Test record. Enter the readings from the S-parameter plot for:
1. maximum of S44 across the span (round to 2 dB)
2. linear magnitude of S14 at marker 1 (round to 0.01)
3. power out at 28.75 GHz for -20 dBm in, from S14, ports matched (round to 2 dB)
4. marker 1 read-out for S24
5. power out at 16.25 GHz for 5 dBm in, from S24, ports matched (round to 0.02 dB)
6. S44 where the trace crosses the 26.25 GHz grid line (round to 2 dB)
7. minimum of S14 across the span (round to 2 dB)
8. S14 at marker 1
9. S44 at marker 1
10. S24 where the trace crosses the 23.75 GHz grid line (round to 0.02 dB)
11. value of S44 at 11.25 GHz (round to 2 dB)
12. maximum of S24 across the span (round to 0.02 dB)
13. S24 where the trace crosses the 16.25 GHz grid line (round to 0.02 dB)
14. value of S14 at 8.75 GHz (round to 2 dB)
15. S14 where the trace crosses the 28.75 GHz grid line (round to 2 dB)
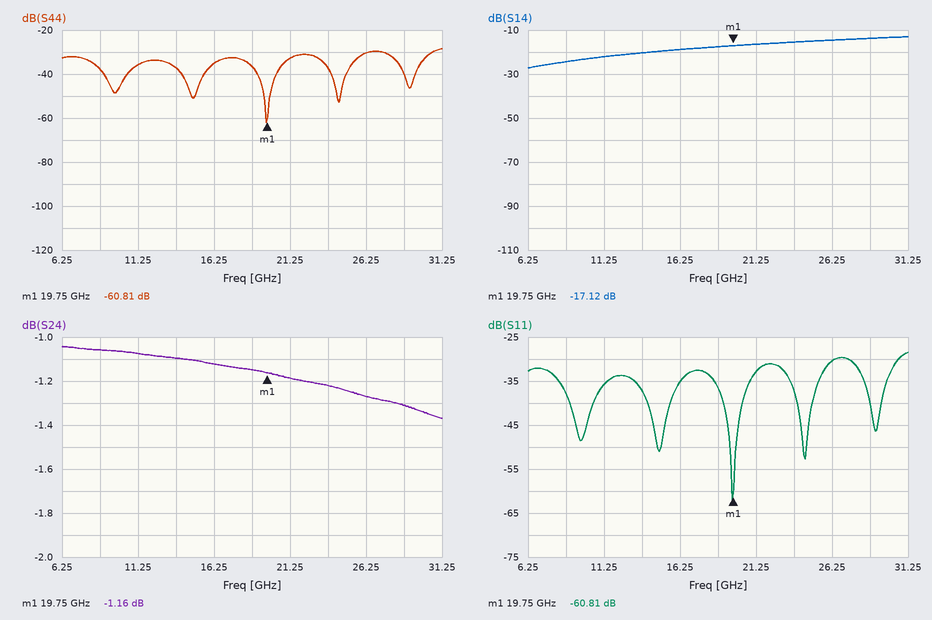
-28 dB
0.14
-34 dBm
-1.16 dB
3.88 dBm
-30 dB
-28 dB
-17.12 dB
-60.81 dB
-1.22 dB
-36 dB
-1.04 dB
-1.12 dB
-24 dB
-14 dB
